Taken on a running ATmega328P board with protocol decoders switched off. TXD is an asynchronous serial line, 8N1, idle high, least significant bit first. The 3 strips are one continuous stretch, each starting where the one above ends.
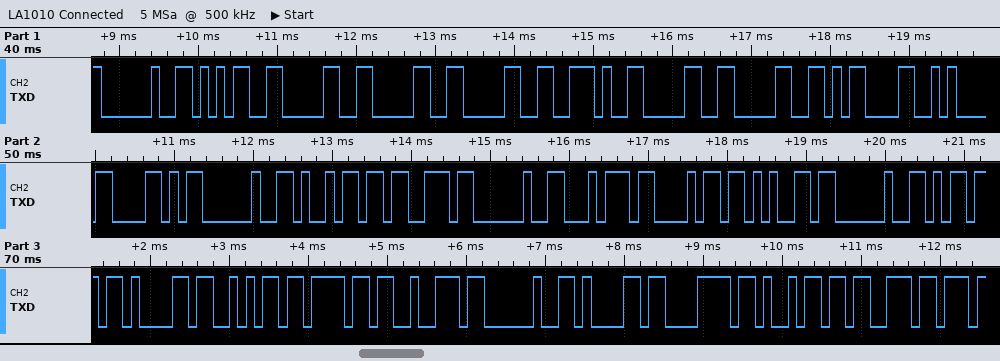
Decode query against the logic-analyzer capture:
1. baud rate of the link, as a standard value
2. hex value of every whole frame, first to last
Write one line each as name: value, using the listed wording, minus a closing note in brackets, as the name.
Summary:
baud rate of the link, as a standard value: 9600 baud
hex value of every whole frame, first to last: 20 35 30 30 30 2E 30 30 0D 0A 58 20 69 73 20 74 68 65 20 6D 61 6A 6F 72 20 61 78 69 73
